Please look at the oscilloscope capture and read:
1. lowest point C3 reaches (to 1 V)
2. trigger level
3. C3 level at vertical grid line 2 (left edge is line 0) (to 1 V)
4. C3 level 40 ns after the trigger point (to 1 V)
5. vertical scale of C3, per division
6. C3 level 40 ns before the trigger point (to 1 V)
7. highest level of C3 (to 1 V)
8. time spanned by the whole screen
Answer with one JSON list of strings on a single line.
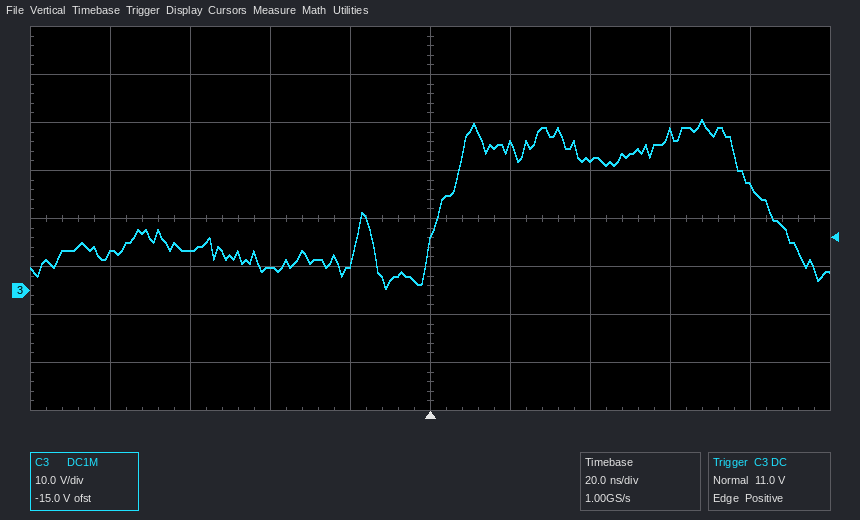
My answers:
["0 V", "11.0 V", "8 V", "27 V", "10 V", "5 V", "36 V", "200 ns"]
